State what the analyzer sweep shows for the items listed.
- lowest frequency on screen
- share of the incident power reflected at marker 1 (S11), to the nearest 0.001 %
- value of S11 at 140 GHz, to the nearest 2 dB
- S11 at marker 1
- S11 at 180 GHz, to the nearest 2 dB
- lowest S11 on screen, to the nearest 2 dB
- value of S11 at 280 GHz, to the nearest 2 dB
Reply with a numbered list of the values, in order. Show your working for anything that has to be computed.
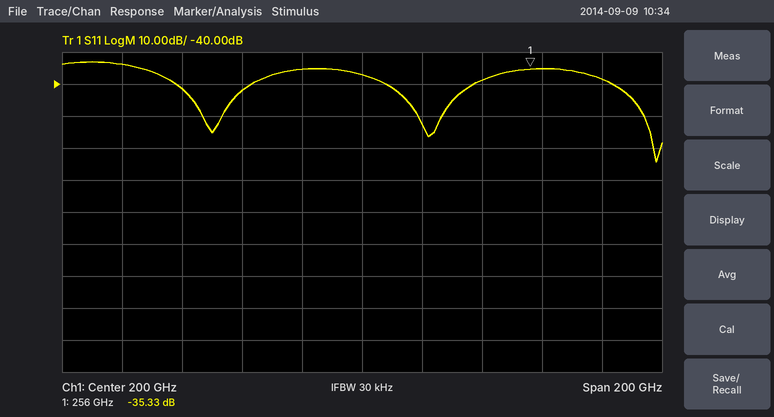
1. 100 GHz
2. 10^(-35.33/10) ≈ 0.029 %
3. -42 dB
4. -35.33 dB
5. -36 dB
6. -64 dB
7. -38 dB
